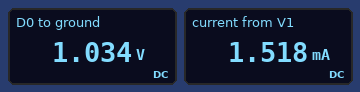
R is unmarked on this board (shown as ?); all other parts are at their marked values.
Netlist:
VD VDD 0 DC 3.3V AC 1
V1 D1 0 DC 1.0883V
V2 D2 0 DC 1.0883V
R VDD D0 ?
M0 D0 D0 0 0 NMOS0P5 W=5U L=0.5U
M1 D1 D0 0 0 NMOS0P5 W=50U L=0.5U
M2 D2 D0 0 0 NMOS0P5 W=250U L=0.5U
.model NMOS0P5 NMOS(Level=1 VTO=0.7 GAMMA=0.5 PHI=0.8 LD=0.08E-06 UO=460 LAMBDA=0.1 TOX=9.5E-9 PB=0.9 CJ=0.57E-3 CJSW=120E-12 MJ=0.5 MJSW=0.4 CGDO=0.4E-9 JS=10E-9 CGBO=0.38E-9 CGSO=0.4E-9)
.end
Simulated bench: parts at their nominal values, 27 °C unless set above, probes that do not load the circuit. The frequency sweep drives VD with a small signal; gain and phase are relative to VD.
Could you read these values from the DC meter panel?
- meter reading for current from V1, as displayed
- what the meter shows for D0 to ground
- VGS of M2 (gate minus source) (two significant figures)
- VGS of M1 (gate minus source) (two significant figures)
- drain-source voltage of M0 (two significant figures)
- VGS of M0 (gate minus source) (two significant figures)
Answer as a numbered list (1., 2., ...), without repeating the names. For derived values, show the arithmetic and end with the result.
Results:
1. 1.518 mA
2. 1.034 V
3. 1.034 V = 1.0 V
4. 1.034 V = 1.0 V
5. 1.034 V = 1.0 V
6. 1.034 V = 1.0 V
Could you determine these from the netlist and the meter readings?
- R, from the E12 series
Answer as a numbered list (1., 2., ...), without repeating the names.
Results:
1. 15 kΩ
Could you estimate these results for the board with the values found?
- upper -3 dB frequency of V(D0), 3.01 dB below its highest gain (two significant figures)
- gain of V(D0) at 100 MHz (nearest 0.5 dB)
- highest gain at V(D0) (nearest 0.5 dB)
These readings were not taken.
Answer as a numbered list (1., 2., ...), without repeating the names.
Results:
1. 320 MHz
2. -24.0 dB
3. -23.5 dB
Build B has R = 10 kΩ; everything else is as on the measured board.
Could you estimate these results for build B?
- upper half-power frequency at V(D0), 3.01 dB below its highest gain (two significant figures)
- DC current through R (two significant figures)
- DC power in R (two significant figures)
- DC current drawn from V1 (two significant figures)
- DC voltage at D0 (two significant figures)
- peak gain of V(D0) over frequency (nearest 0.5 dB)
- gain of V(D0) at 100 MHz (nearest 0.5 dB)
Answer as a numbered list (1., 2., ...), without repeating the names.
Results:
1. 390 MHz
2. 220 µA
3. 480 µW
4. 2.2 mA
5. 1.1 V
6. -21.5 dB
7. -22.0 dB
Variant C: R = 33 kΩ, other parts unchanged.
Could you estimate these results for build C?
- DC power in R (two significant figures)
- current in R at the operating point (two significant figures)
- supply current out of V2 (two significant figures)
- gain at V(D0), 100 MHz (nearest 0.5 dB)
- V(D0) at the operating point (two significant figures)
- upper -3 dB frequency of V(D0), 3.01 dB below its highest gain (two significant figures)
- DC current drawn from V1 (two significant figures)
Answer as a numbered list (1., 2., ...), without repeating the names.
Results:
1. 170 µW
2. 72 µA
3. 3.6 mA
4. -27.5 dB
5. 930 mV
6. 210 MHz
7. 730 µA
